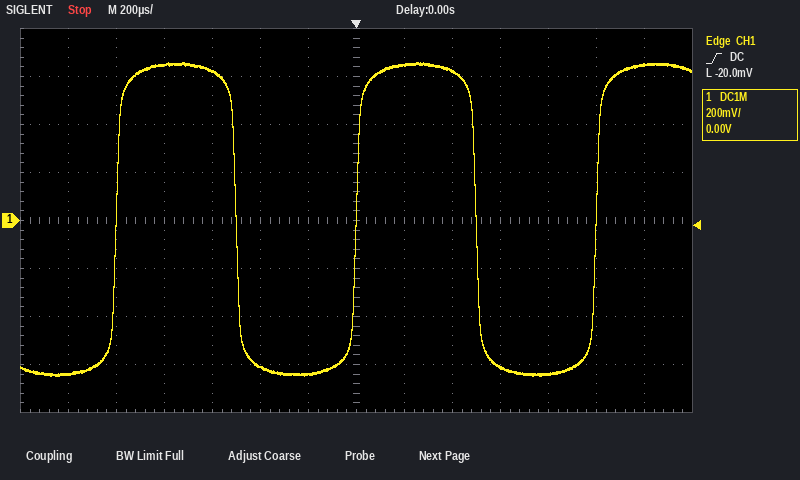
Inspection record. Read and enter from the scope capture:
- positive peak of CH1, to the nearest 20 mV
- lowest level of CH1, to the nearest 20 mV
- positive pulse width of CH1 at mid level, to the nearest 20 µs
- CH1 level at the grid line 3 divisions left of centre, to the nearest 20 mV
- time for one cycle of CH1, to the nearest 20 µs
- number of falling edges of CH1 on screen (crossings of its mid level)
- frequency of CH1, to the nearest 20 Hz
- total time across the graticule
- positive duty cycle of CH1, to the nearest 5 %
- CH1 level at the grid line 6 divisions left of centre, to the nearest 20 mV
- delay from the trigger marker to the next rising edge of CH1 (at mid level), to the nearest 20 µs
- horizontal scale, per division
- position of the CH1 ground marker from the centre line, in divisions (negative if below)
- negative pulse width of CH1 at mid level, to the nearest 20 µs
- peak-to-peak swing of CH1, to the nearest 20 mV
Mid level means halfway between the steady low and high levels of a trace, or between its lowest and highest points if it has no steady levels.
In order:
660 mV
-640 mV
500 µs
620 mV
1.00 ms
2
1.00 kHz
2.8 ms
50 %
-640 mV
1.00 ms
200 µs
0.0 div
500 µs
1.30 V
